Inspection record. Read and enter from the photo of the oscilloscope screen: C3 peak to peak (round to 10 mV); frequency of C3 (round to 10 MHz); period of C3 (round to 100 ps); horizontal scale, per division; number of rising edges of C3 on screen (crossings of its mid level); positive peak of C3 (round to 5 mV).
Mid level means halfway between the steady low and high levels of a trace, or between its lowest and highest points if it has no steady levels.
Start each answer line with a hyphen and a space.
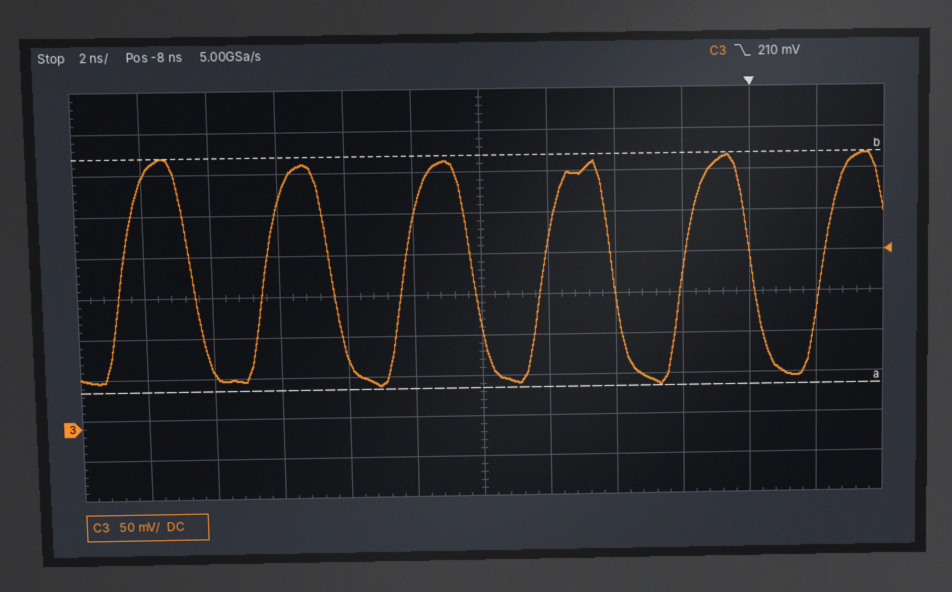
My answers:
- 280 mV
- 240 MHz
- 4.2 ns
- 2 ns
- 6
- 330 mV
